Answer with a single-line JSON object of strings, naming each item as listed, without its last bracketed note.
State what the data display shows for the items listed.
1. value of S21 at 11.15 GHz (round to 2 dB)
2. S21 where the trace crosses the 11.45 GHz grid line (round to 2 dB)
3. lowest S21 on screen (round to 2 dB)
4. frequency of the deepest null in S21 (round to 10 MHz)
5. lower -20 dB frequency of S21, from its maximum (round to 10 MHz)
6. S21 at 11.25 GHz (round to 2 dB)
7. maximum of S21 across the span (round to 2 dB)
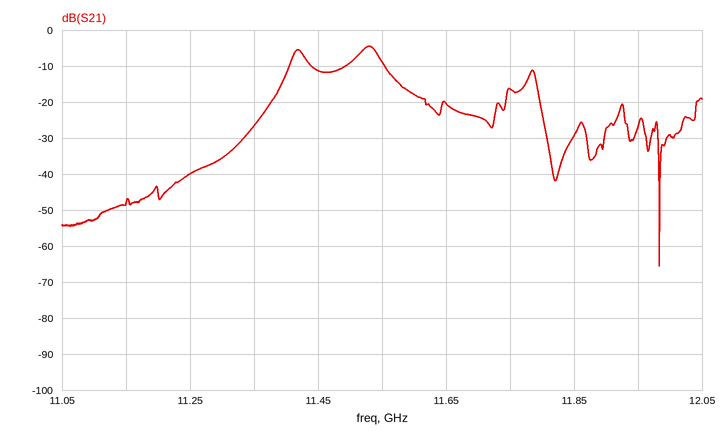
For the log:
{"value of S21 at 11.15 GHz": "-48 dB", "S21 where the trace crosses the 11.45 GHz grid line": "-12 dB", "lowest S21 on screen": "-66 dB", "frequency of the deepest null in S21": "11.98 GHz", "lower -20 dB frequency of S21, from its maximum": "11.36 GHz", "S21 at 11.25 GHz": "-40 dB", "maximum of S21 across the span": "-4 dB"}
